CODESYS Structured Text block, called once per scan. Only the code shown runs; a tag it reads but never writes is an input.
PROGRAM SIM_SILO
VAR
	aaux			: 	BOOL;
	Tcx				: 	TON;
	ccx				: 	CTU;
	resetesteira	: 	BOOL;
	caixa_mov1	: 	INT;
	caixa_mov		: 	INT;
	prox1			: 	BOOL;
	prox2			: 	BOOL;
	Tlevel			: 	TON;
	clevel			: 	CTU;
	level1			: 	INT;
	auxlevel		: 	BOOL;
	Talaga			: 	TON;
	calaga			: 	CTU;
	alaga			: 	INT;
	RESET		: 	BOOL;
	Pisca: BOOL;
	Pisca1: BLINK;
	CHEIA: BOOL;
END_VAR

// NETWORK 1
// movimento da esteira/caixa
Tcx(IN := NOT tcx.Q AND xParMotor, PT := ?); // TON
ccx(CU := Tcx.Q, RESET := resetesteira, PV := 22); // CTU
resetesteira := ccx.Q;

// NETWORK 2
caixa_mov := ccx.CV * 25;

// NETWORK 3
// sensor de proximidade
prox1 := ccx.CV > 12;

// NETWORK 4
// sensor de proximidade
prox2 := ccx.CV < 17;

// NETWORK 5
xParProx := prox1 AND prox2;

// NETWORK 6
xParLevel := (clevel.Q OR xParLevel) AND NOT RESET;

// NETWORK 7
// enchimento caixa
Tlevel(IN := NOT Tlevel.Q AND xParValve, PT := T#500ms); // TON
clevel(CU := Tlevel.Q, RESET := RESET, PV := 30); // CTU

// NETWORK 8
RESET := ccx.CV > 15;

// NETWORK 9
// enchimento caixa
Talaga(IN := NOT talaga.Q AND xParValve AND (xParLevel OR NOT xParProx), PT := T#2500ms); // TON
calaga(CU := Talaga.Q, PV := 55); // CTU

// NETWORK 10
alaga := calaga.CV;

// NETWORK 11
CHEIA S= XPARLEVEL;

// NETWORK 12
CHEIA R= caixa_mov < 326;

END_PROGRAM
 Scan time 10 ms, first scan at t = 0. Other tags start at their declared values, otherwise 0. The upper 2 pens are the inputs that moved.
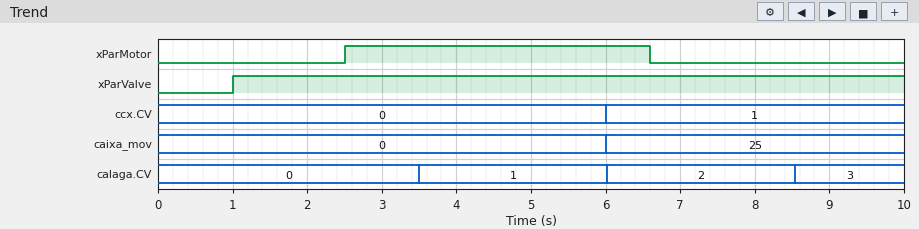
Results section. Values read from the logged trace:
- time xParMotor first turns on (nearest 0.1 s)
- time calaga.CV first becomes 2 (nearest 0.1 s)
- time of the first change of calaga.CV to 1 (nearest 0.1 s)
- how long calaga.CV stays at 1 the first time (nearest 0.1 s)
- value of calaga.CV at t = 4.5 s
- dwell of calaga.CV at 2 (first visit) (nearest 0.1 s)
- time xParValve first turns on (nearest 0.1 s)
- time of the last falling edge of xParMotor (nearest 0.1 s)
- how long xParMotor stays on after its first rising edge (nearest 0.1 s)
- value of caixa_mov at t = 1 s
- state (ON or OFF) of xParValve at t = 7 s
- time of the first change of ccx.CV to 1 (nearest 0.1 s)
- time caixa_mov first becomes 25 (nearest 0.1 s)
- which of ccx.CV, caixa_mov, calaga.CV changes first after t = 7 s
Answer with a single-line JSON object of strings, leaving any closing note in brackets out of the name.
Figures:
{"time xParMotor first turns on": "2.5 s", "time calaga.CV first becomes 2": "6.0 s", "time of the first change of calaga.CV to 1": "3.5 s", "how long calaga.CV stays at 1 the first time": "2.5 s", "value of calaga.CV at t = 4.5 s": "1", "dwell of calaga.CV at 2 (first visit)": "2.5 s", "time xParValve first turns on": "1.0 s", "time of the last falling edge of xParMotor": "6.6 s", "how long xParMotor stays on after its first rising edge": "4.1 s", "value of caixa_mov at t = 1 s": "0", "state (ON or OFF) of xParValve at t = 7 s": "ON", "time of the first change of ccx.CV to 1": "6.0 s", "time caixa_mov first becomes 25": "6.0 s", "which of ccx.CV, caixa_mov, calaga.CV changes first after t = 7 s": "calaga.CV"}
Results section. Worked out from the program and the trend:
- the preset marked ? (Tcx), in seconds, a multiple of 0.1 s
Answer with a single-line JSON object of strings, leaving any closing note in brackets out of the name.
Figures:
{"the preset marked ? (Tcx), in seconds, a multiple of 0.1 s": "3.5 s"}
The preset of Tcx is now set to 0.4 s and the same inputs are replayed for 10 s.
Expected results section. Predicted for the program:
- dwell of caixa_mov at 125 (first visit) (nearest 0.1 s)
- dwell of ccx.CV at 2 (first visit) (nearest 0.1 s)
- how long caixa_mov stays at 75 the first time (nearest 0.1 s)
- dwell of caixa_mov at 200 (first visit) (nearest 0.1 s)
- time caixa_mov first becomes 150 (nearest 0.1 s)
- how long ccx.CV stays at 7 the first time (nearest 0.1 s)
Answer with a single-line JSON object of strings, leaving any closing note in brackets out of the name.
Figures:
{"dwell of caixa_mov at 125 (first visit)": "0.4 s", "dwell of ccx.CV at 2 (first visit)": "0.4 s", "how long caixa_mov stays at 75 the first time": "0.4 s", "dwell of caixa_mov at 200 (first visit)": "0.4 s", "time caixa_mov first becomes 150": "5.0 s", "how long ccx.CV stays at 7 the first time": "0.4 s"}
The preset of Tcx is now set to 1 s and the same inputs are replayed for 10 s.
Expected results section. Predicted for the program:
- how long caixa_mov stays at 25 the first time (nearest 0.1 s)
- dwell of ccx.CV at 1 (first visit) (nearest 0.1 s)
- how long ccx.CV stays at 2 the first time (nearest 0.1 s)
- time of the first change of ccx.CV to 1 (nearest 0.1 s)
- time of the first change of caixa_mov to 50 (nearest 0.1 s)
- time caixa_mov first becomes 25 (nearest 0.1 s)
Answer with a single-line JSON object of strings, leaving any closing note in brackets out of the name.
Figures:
{"how long caixa_mov stays at 25 the first time": "1.0 s", "dwell of ccx.CV at 1 (first visit)": "1.0 s", "how long ccx.CV stays at 2 the first time": "1.0 s", "time of the first change of ccx.CV to 1": "3.5 s", "time of the first change of caixa_mov to 50": "4.5 s", "time caixa_mov first becomes 25": "3.5 s"}
